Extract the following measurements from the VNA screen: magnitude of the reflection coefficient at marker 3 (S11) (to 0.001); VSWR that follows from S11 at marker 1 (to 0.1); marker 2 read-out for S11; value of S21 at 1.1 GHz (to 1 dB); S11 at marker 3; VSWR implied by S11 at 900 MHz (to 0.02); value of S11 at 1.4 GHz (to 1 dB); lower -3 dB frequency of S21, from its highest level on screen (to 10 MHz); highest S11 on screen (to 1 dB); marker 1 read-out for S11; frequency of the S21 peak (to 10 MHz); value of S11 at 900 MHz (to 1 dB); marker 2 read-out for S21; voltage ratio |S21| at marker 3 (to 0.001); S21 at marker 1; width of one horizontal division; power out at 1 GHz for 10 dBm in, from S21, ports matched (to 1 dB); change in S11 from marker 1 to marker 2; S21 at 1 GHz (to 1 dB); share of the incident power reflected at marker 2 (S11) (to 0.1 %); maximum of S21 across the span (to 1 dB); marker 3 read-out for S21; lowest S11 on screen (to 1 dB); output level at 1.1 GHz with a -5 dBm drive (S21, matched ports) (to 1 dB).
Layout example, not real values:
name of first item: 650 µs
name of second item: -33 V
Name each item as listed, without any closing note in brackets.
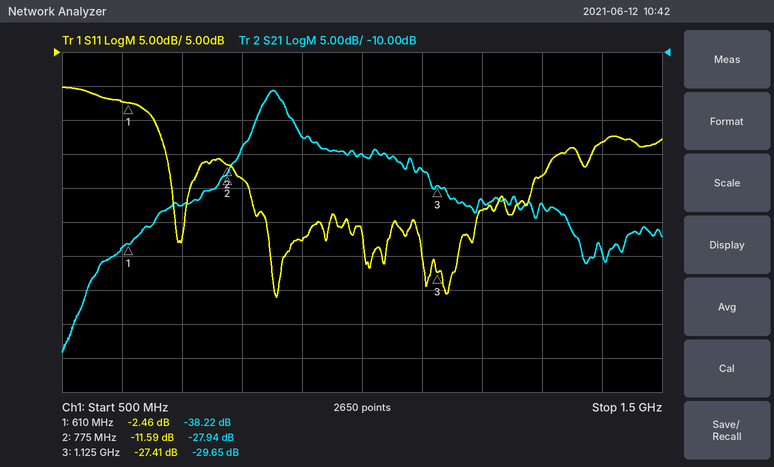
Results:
magnitude of the reflection coefficient at marker 3 (S11): 0.043
VSWR that follows from S11 at marker 1: 7.1
marker 2 read-out for S11: -11.59 dB
value of S21 at 1.1 GHz: -27 dB
S11 at marker 3: -27.41 dB
VSWR implied by S11 at 900 MHz: 1.16
value of S11 at 1.4 GHz: -8 dB
lower -3 dB frequency of S21, from its highest level on screen: 830 MHz
highest S11 on screen: 0 dB
marker 1 read-out for S11: -2.46 dB
frequency of the S21 peak: 850 MHz
value of S11 at 900 MHz: -23 dB
marker 2 read-out for S21: -27.94 dB
voltage ratio |S21| at marker 3: 0.033
S21 at marker 1: -38.22 dB
width of one horizontal division: 100 MHz
power out at 1 GHz for 10 dBm in, from S21, ports matched: -15 dBm
change in S11 from marker 1 to marker 2: -9.13 dB
S21 at 1 GHz: -25 dB
share of the incident power reflected at marker 2 (S11): 6.9 %
maximum of S21 across the span: -16 dB
marker 3 read-out for S21: -29.65 dB
lowest S11 on screen: -31 dB
output level at 1.1 GHz with a -5 dBm drive (S21, matched ports): -32 dBm
